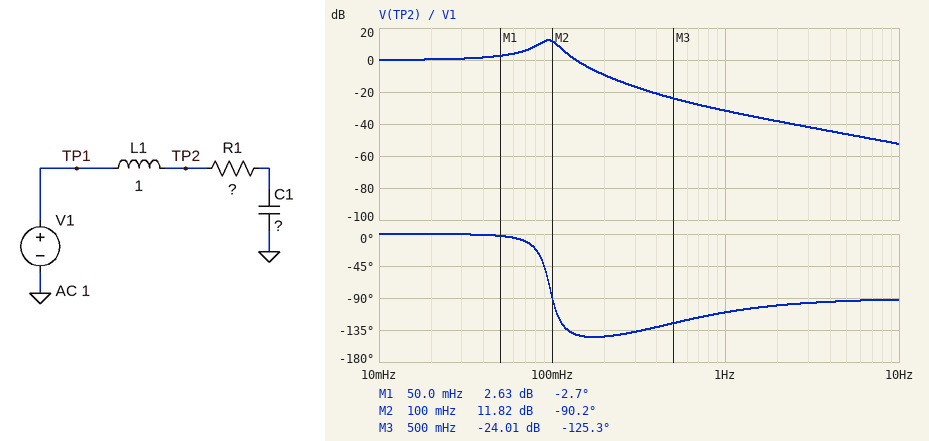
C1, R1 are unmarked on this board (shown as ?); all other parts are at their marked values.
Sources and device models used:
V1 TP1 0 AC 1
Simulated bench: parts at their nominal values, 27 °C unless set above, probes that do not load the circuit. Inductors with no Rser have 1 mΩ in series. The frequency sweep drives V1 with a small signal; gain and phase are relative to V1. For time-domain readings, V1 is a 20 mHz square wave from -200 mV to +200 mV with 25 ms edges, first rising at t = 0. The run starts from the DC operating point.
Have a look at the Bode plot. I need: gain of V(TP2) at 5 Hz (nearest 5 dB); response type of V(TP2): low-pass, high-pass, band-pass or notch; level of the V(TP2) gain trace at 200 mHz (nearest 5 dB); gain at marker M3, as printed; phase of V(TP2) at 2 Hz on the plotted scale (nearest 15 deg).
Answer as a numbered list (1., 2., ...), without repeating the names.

1. -45 dB
2. low-pass
3. -10 dB
4. -24.01 dB
5. -105 deg
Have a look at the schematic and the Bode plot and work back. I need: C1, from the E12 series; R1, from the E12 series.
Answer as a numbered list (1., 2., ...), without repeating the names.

1. 2.7 F
2. 0.15 Ω
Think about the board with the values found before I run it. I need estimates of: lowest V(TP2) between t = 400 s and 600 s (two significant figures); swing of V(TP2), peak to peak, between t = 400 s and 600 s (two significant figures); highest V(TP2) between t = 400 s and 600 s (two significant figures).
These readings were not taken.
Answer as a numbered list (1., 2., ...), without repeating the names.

1. -510 mV
2. 1.0 V
3. 510 mV
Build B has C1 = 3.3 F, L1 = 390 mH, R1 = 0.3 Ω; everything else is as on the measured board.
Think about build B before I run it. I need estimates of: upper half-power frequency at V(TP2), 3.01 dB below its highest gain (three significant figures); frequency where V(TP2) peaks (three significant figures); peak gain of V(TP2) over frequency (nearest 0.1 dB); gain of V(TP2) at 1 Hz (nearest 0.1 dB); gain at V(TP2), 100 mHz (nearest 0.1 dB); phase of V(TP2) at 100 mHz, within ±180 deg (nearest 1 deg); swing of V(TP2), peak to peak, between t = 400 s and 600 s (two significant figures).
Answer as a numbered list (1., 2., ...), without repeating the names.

1. 185 mHz
2. 123 mHz
3. 3.9 dB
4. -18.0 dB
5. 3.4 dB
6. -20 deg
7. 670 mV
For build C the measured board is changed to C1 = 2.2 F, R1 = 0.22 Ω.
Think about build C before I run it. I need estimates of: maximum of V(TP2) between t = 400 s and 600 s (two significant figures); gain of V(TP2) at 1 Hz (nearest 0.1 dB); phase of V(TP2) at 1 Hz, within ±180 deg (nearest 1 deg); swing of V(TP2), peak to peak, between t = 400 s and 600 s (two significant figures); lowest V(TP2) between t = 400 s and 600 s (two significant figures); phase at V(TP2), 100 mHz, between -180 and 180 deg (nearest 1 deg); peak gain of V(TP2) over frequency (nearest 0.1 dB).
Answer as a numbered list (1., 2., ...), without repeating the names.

1. 460 mV
2. -28.6 dB
3. -106 deg
4. 930 mV
5. -460 mV
6. -50 deg
7. 10.2 dB
